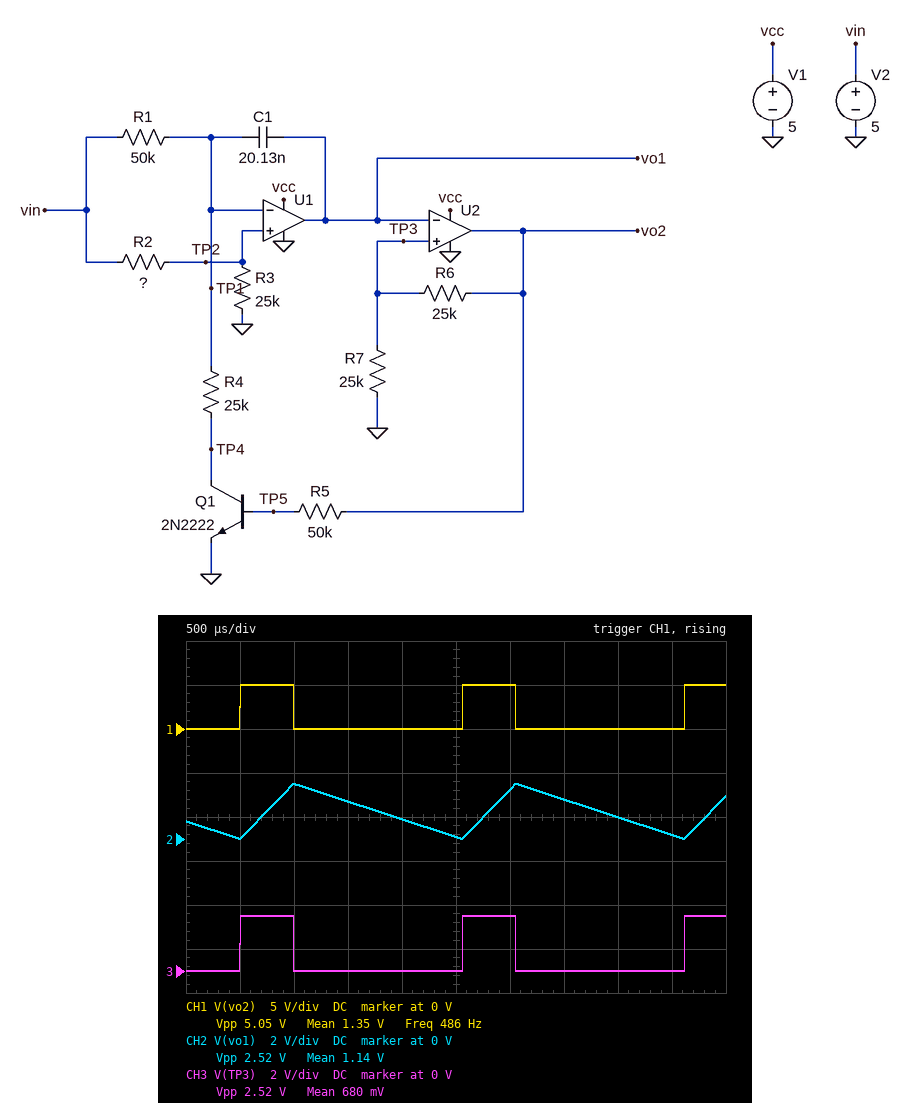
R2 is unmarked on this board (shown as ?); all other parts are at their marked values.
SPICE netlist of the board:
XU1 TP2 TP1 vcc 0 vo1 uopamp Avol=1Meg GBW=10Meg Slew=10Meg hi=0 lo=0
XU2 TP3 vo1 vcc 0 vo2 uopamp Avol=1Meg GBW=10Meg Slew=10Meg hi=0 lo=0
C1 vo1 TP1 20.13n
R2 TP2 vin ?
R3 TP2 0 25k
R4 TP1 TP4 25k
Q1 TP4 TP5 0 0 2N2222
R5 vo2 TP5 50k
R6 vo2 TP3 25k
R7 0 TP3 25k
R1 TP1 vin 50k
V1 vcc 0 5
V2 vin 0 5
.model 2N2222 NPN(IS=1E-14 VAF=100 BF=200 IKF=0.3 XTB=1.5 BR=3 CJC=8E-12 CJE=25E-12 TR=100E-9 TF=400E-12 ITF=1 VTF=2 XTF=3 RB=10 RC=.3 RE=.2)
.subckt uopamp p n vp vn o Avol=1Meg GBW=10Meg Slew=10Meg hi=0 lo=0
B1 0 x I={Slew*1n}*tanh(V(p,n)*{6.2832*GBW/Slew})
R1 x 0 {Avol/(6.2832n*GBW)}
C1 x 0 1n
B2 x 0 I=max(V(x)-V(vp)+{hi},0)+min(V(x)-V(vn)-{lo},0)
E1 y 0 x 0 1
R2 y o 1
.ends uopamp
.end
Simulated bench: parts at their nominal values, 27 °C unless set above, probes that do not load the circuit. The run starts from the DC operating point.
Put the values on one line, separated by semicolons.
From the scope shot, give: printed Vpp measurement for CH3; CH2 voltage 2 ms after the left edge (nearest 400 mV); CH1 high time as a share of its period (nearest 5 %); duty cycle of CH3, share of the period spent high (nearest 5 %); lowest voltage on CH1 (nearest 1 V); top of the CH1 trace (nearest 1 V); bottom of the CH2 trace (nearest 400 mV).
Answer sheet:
2.52 V; 800 mV; 25 %; 25 %; 0 V; 5 V; 0 V
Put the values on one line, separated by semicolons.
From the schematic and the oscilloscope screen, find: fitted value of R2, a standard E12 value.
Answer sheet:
12 kΩ
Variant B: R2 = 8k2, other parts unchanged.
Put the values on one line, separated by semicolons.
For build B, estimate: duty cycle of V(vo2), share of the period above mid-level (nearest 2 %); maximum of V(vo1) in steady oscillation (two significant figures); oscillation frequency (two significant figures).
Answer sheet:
16 %; 2.5 V; 410 Hz
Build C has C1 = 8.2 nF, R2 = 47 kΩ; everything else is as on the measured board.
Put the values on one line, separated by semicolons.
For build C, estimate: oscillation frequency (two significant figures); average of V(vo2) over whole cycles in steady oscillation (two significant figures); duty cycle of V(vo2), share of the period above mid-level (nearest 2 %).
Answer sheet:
170 Hz; 4.7 V; 94 %
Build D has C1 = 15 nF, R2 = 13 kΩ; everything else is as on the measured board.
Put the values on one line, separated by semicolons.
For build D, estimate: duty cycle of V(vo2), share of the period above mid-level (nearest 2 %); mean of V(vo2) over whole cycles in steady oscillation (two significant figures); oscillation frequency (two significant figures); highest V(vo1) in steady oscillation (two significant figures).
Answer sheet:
26 %; 1.3 V; 670 Hz; 2.5 V
